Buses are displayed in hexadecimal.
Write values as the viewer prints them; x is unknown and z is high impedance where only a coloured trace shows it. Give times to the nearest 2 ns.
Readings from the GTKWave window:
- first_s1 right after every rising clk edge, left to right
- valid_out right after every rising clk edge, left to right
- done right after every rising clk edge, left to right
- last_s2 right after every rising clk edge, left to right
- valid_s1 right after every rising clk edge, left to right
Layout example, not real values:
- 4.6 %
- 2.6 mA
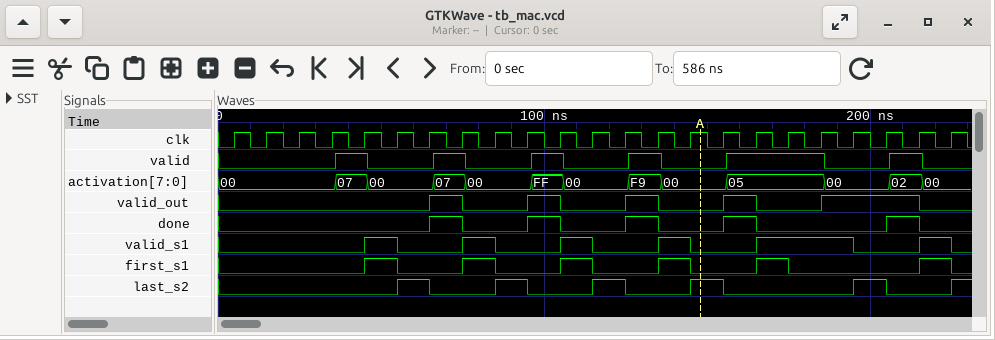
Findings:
- 0 0 0 0 1 0 0 1 0 0 1 0 0 1 0 0 1 0 0 0 0 1 0
- 0 0 0 0 0 0 1 0 0 1 0 0 1 0 0 1 0 0 1 1 1 0 0
- 0 0 0 0 0 0 1 0 0 1 0 0 1 0 0 1 0 0 0 0 1 0 0
- 0 0 0 0 0 1 0 0 1 0 0 1 0 0 1 0 0 0 0 1 0 0 1
- 0 0 0 0 1 0 0 1 0 0 1 0 0 1 0 0 1 1 1 0 0 1 0
